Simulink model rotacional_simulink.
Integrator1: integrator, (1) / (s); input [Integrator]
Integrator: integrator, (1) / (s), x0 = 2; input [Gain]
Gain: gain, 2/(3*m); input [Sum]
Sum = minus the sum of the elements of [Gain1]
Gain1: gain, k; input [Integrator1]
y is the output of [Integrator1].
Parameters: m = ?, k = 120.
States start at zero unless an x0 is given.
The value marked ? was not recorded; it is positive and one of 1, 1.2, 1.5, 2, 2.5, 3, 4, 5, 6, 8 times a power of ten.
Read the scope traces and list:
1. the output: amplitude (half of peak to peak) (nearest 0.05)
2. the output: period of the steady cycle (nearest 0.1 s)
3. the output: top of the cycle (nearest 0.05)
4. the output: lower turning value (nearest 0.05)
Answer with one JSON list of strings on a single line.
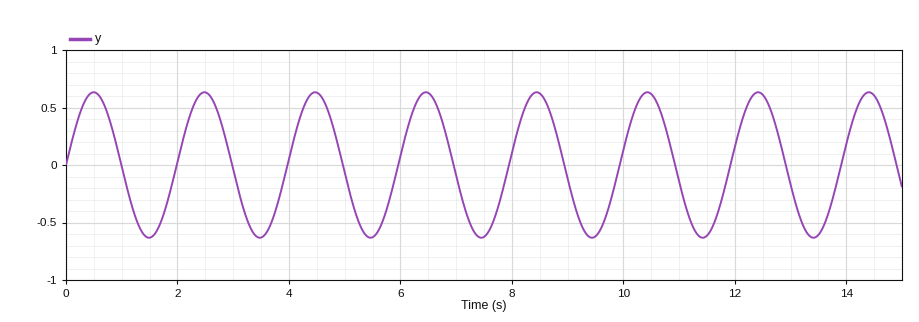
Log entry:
["0.65", "2.0 s", "0.65", "-0.65"]
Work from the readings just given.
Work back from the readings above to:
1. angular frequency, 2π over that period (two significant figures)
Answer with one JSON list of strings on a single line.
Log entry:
["3.1 rad/s"]
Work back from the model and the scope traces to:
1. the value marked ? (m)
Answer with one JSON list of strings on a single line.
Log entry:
["8"]
